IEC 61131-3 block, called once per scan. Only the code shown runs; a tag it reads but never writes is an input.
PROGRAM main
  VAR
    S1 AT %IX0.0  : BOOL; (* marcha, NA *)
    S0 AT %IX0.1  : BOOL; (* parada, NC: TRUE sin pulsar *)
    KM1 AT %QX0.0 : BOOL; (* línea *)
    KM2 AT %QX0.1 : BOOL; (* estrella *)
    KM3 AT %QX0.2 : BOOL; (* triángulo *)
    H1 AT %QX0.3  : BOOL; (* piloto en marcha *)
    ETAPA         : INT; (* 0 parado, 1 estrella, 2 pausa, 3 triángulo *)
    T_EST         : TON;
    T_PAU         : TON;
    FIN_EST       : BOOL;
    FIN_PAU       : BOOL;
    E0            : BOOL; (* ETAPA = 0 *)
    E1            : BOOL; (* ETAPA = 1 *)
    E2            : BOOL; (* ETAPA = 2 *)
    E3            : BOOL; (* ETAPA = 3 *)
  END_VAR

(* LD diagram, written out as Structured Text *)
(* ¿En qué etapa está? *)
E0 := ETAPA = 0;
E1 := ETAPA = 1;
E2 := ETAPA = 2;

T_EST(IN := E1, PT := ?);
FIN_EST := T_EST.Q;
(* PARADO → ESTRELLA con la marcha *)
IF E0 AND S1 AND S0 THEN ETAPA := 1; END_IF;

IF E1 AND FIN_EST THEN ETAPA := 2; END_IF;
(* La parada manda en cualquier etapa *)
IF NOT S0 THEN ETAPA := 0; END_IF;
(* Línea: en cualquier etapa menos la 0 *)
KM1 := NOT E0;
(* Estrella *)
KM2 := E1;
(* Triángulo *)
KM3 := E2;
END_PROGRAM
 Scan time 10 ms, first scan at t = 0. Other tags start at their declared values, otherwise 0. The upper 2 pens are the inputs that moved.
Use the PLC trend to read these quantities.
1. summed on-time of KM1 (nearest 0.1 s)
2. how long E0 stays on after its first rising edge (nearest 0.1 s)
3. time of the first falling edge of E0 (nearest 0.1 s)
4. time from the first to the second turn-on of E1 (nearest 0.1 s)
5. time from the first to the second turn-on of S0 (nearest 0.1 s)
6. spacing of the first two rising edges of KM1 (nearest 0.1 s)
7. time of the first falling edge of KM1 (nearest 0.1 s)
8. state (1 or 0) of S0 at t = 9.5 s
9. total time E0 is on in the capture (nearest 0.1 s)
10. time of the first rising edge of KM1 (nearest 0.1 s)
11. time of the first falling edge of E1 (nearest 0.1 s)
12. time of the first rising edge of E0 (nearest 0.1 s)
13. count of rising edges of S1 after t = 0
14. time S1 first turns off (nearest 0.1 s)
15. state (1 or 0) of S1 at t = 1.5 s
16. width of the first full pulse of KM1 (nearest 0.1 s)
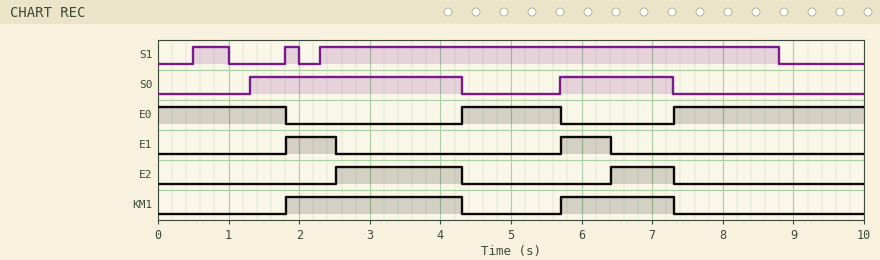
4.1 s
1.4 s
1.8 s
3.9 s
4.4 s
3.9 s
4.3 s
0
5.9 s
1.8 s
2.5 s
4.3 s
3
1.0 s
0
2.5 s
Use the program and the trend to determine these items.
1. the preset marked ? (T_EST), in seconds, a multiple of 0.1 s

0.7 s
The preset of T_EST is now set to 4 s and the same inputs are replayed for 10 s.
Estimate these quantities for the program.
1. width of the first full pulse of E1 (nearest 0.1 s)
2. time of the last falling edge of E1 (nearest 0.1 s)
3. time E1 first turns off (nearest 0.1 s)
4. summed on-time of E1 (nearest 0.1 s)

2.5 s
7.3 s
4.3 s
4.1 s
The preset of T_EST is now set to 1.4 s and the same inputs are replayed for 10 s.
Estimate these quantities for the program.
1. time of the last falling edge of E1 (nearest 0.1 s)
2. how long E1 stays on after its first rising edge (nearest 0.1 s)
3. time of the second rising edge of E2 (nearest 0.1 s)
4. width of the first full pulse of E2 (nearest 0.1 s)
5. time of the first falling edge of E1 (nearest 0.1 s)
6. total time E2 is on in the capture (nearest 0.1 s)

7.1 s
1.4 s
7.1 s
1.1 s
3.2 s
1.3 s
